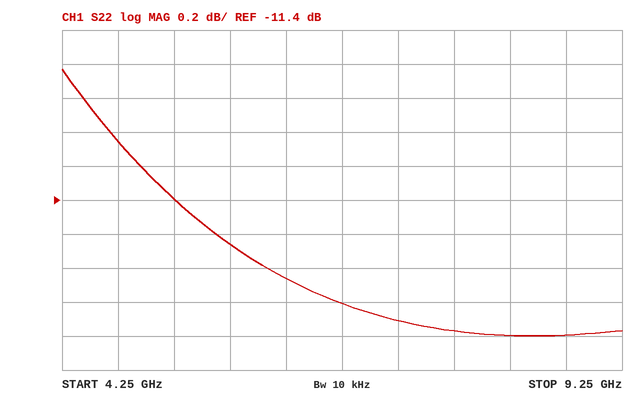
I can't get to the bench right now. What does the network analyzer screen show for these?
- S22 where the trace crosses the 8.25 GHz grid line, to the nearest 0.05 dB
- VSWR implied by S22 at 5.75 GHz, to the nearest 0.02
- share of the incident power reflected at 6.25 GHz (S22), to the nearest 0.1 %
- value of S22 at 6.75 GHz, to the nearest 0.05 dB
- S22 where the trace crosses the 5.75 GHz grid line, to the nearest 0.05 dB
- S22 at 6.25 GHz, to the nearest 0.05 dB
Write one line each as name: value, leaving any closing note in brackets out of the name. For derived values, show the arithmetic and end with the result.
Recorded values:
S22 where the trace crosses the 8.25 GHz grid line, to the nearest 0.05 dB: -12.20 dB
VSWR implied by S22 at 5.75 GHz, to the nearest 0.02: |Γ| = 10^(-11.65/20) = 0.2615; VSWR = (1 + 0.2615)/(1 − 0.2615) ≈ 1.71, so 1.70 to the nearest 0.02
share of the incident power reflected at 6.25 GHz (S22), to the nearest 0.1 %: 10^(-11.85/10) ≈ 6.5 %
value of S22 at 6.75 GHz, to the nearest 0.05 dB: -12.00 dB
S22 where the trace crosses the 5.75 GHz grid line, to the nearest 0.05 dB: -11.65 dB
S22 at 6.25 GHz, to the nearest 0.05 dB: -11.85 dB
